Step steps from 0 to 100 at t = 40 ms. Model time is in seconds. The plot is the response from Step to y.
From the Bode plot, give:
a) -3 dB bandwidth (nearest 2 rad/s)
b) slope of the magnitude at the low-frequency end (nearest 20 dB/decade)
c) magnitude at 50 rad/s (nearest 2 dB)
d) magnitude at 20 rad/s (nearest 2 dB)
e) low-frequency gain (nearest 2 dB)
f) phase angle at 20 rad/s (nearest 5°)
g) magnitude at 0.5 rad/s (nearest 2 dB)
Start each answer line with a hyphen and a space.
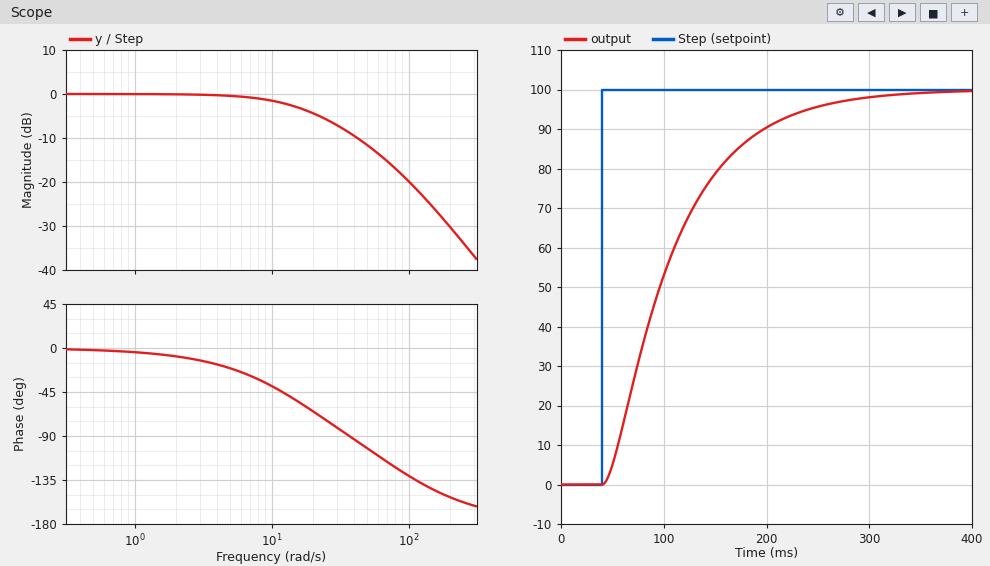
- 16 rad/s
- 0 dB/decade
- -12 dB
- -4 dB
- 0 dB
- -65°
- 0 dB
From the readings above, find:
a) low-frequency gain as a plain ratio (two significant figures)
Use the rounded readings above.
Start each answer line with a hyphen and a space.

- 1.0
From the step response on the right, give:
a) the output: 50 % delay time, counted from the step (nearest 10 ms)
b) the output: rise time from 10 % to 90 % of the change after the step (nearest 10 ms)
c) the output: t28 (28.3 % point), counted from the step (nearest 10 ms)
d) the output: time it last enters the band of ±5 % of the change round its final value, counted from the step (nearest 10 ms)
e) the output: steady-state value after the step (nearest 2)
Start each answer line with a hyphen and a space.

- 60 ms
- 140 ms
- 30 ms
- 200 ms
- 100
